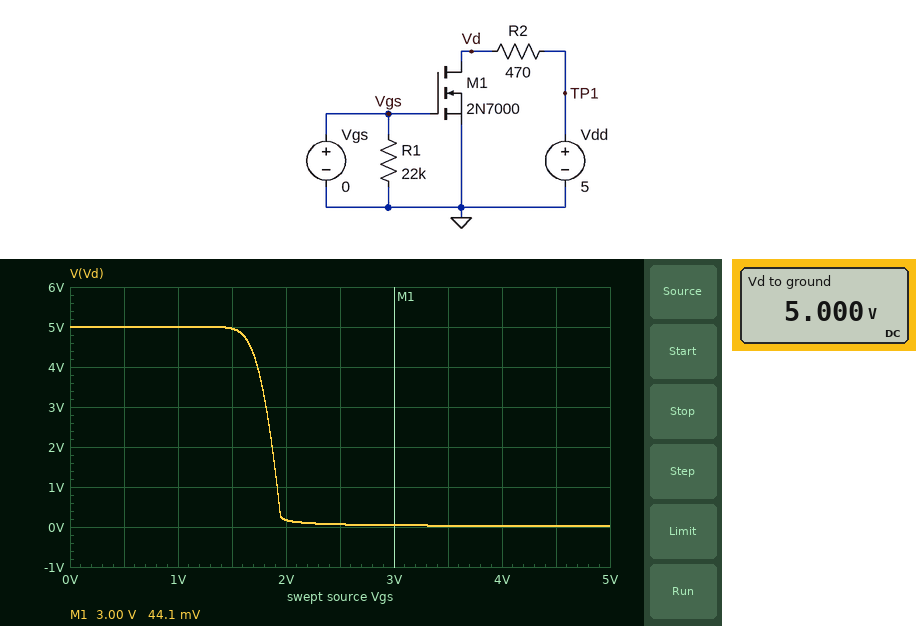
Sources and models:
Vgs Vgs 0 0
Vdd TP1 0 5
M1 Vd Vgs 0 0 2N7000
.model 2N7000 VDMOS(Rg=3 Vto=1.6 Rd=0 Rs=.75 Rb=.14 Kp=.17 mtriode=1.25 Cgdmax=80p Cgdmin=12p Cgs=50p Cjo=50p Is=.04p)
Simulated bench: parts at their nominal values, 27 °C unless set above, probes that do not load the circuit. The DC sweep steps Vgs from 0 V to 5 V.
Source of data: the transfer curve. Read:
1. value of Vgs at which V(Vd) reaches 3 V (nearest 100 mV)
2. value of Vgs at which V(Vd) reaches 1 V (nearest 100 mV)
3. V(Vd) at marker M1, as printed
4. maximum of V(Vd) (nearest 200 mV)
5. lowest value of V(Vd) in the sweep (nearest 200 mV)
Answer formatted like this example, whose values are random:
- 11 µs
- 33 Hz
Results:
- 1.8 V
- 1.9 V
- 44.1 mV
- 5.0 V
- 0 V
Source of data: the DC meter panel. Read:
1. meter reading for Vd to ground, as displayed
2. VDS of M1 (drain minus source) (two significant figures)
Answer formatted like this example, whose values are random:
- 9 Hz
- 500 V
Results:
- 5.000 V
- 5.0 V
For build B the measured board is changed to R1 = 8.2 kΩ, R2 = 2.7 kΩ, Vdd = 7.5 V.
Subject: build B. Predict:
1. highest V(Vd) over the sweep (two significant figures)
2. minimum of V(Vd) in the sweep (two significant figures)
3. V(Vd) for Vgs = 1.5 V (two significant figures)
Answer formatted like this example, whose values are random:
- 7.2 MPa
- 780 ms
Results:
- 7.5 V
- 5.9 mV
- 7.3 V
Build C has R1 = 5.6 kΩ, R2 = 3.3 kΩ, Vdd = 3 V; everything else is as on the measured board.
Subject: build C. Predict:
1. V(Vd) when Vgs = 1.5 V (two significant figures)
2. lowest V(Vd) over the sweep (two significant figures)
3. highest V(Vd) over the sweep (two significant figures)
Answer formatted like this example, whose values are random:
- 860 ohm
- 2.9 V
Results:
- 2.7 V
- 1.9 mV
- 3.0 V
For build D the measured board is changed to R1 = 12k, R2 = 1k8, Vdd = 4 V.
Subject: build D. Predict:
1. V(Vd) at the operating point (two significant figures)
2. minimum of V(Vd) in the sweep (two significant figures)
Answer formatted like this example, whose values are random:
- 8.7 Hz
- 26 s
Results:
- 4.0 V
- 4.7 mV
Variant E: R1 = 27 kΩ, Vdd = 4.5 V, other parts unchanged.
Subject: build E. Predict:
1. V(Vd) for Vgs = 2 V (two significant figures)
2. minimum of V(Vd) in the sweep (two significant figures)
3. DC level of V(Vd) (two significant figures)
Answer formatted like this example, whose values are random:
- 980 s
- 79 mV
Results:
- 150 mV
- 20 mV
- 4.5 V
